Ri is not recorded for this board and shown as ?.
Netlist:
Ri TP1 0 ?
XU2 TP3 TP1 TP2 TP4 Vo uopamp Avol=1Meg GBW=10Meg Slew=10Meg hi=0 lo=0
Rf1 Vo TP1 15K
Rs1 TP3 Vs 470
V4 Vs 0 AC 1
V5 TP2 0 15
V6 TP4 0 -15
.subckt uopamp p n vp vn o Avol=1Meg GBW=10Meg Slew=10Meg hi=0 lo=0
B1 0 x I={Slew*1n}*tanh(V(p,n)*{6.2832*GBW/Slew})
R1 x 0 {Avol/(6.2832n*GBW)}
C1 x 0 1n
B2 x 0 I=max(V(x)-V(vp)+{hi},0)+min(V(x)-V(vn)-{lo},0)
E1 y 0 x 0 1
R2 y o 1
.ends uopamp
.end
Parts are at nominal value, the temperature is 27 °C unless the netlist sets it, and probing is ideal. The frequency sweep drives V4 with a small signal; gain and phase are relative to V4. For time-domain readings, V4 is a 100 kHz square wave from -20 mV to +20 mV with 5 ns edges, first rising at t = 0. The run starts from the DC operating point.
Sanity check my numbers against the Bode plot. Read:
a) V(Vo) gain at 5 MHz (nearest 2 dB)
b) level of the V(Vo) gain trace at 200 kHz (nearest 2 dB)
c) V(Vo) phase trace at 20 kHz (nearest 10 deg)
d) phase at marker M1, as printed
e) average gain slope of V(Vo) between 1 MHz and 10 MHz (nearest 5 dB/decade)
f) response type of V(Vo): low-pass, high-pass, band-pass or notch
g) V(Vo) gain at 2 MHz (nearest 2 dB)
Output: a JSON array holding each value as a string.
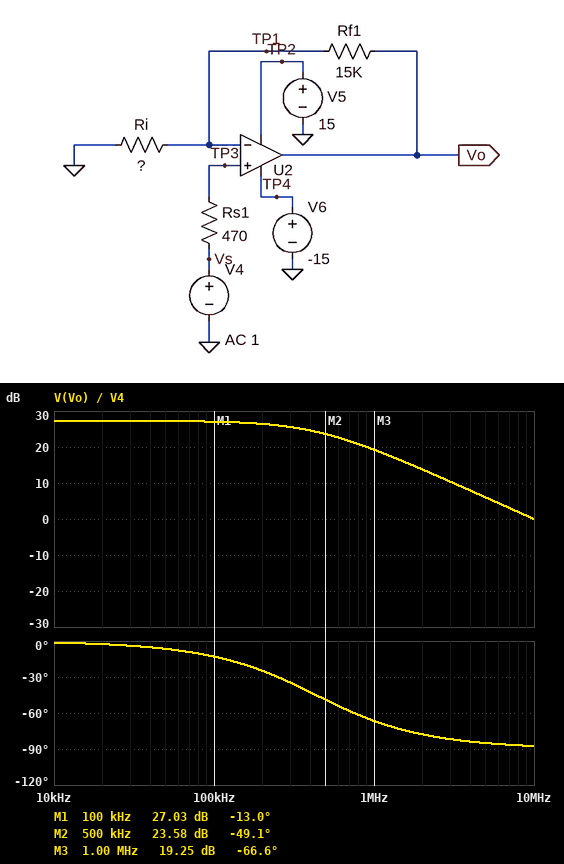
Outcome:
["6 dB", "26 dB", "0 deg", "-13.0 deg", "-20 dB/decade", "low-pass", "14 dB"]
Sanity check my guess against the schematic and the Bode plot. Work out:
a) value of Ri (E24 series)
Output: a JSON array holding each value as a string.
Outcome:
["680 Ω"]
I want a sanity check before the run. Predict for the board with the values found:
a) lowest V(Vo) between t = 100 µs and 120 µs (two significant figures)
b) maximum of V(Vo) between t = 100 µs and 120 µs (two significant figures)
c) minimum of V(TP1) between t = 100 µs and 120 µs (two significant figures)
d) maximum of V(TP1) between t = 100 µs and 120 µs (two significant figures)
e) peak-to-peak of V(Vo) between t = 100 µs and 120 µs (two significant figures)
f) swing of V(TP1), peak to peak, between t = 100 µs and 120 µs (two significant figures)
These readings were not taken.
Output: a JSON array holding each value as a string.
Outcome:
["-460 mV", "460 mV", "-20 mV", "20 mV", "920 mV", "40 mV"]
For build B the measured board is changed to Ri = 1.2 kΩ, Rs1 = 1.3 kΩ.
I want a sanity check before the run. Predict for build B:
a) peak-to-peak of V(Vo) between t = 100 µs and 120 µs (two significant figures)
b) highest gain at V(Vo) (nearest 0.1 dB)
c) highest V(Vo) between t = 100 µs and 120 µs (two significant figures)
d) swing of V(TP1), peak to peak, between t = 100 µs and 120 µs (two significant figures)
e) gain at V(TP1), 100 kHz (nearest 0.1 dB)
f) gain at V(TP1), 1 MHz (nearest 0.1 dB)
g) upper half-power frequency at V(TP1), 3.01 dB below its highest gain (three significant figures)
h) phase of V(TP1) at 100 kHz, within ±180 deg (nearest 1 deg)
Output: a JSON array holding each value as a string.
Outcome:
["540 mV", "22.6 dB", "270 mV", "40 mV", "-0.1 dB", "-4.5 dB", "741 kHz", "-8 deg"]
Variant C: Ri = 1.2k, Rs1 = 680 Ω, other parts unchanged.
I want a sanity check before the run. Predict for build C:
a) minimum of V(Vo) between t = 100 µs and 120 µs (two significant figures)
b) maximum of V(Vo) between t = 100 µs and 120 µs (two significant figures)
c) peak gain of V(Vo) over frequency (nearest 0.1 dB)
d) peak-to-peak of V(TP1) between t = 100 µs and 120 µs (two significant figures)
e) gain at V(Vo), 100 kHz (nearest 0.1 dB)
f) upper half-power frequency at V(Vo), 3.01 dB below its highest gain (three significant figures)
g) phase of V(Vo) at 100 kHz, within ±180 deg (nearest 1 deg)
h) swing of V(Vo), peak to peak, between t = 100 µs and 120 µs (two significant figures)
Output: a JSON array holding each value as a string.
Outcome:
["-270 mV", "270 mV", "22.6 dB", "40 mV", "22.5 dB", "741 kHz", "-8 deg", "540 mV"]
